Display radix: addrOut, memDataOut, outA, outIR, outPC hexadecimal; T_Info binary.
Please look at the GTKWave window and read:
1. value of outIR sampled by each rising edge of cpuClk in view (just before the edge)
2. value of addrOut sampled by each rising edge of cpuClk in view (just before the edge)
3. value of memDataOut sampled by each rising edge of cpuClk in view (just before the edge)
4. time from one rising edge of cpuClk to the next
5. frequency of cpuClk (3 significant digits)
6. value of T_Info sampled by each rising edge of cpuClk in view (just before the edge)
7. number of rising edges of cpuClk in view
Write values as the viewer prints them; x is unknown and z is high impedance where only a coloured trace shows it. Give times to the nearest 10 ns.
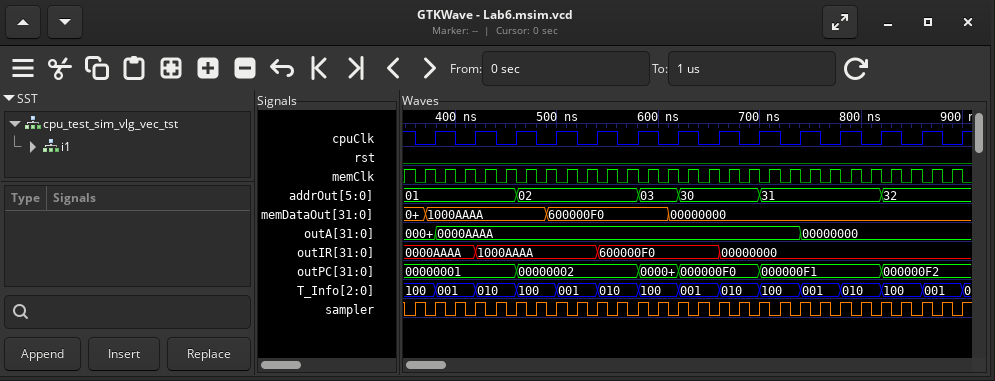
0000AAAA, 0000AAAA, 1000AAAA, 1000AAAA, 1000AAAA, 600000F0, 600000F0, 600000F0, 00000000, 00000000, 00000000, 00000000, 00000000, 00000000
01, 01, 01, 02, 02, 02, 03, 30, 30, 31, 31, 31, 32, 32
1000AAAA, 1000AAAA, 1000AAAA, 600000F0, 600000F0, 600000F0, 00000000, 00000000, 00000000, 00000000, 00000000, 00000000, 00000000, 00000000
40 ns
25.0 MHz
100, 001, 010, 100, 001, 010, 100, 001, 010, 100, 001, 010, 100, 001
14
